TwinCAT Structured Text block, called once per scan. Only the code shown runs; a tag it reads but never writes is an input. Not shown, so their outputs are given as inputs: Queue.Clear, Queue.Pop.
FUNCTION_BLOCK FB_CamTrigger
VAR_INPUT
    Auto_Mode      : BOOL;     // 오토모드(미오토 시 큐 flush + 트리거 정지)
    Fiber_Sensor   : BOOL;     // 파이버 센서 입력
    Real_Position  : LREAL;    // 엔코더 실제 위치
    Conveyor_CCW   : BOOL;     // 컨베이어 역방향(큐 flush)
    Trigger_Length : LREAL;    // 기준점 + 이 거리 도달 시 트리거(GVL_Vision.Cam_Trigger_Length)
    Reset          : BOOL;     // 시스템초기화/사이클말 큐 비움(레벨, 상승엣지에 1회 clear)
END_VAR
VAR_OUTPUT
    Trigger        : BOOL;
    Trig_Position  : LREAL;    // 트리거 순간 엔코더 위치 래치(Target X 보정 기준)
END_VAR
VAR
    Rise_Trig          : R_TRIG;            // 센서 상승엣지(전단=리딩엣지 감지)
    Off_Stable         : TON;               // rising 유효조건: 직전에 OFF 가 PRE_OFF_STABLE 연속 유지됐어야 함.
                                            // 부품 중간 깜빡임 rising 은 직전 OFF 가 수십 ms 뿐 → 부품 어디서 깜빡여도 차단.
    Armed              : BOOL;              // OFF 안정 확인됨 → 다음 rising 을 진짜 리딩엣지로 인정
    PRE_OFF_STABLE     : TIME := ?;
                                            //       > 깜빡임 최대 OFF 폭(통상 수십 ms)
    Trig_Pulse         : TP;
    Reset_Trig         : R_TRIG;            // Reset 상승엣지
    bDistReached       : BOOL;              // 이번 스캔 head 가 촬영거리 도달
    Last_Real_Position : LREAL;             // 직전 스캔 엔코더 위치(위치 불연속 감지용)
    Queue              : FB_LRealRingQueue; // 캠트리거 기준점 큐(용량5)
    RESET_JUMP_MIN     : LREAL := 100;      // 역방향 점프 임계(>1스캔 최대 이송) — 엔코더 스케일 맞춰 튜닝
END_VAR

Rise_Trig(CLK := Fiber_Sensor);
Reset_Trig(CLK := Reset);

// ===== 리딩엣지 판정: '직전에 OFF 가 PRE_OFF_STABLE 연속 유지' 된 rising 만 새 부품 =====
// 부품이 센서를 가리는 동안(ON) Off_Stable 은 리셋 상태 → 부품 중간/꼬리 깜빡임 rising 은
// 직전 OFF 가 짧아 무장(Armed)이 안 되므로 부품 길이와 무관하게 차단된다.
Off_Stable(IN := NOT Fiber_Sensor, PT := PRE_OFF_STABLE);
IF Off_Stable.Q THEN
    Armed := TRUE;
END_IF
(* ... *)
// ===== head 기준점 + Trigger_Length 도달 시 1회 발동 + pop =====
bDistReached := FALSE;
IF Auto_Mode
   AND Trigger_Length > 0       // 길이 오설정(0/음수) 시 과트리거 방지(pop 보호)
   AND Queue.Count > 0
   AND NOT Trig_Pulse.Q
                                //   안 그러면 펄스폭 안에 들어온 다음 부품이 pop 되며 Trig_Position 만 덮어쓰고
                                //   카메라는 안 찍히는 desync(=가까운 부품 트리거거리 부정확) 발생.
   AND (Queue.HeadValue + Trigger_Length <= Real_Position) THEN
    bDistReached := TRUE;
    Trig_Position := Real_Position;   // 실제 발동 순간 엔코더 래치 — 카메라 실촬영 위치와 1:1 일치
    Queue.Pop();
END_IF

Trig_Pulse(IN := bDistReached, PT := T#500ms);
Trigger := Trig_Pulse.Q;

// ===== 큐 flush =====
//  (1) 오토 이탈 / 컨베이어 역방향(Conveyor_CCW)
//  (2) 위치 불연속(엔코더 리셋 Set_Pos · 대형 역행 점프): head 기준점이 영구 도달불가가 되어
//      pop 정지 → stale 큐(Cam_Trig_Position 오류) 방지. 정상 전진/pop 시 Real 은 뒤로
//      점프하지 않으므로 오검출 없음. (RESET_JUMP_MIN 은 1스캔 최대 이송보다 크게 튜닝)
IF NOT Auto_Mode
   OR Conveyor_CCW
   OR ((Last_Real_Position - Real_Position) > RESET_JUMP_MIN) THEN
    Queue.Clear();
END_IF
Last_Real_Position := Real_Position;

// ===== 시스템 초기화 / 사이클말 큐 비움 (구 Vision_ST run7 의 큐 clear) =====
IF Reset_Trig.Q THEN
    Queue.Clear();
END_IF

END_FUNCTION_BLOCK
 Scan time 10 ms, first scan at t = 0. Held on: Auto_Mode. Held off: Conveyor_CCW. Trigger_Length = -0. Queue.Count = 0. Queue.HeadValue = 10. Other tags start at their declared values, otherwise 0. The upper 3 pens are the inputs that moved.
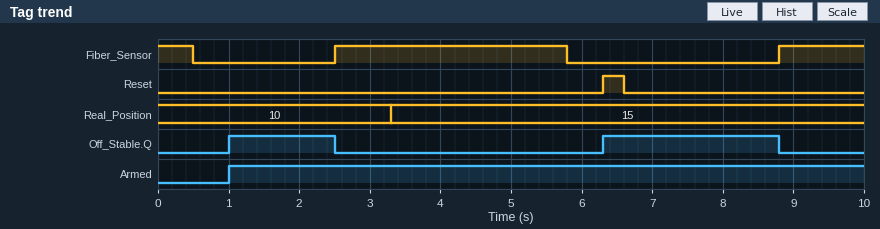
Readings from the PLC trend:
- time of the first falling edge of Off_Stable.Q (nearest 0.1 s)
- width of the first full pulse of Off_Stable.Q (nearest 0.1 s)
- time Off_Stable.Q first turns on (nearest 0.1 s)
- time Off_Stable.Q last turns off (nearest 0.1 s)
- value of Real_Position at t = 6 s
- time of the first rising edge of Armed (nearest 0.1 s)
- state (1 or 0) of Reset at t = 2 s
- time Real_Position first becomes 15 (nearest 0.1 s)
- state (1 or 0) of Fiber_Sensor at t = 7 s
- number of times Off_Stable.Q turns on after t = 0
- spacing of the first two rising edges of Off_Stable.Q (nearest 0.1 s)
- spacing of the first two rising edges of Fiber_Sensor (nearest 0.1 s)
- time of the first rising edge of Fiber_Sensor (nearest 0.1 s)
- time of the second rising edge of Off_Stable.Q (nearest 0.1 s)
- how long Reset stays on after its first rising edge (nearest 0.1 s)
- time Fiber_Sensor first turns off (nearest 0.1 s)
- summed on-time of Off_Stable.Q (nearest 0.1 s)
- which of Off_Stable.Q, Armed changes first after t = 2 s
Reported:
2.5 s
1.5 s
1.0 s
8.8 s
15
1.0 s
0
3.3 s
0
2
5.3 s
6.3 s
2.5 s
6.3 s
0.3 s
0.5 s
4.0 s
Off_Stable.Q
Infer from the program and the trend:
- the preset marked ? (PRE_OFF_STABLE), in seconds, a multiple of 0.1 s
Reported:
0.5 s
